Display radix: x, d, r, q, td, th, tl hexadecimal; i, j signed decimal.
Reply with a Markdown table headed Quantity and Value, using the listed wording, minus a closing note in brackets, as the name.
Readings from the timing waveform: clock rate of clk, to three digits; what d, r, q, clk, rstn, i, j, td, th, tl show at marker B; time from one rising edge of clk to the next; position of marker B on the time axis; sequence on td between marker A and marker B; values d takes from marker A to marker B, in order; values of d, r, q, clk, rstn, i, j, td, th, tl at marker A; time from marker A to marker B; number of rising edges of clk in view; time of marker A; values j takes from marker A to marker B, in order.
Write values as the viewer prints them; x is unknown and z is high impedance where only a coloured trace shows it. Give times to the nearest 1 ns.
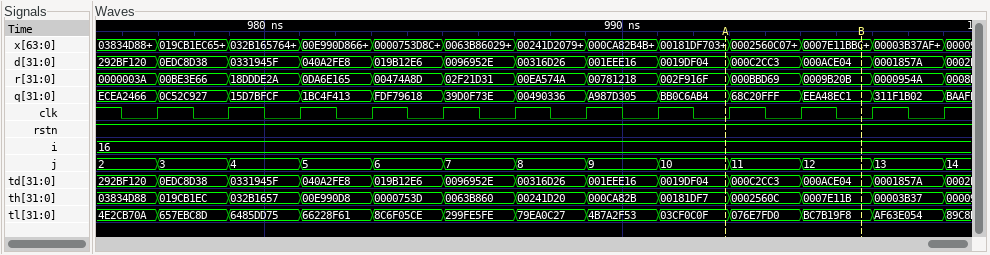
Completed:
| Quantity | Value |
|---|---|
| clock rate of clk, to three digits | 500 MHz |
| what d, r, q, clk, rstn, i, j, td, th, tl show at marker B | d=000ACE04, r=0009B20B, q=EEA48EC1, clk=0, rstn=1, i=16, j=12, td=000ACE04, th=0007E11B, tl=BC7B19F8 |
| time from one rising edge of clk to the next | 2 ns |
| position of marker B on the time axis | 997 ns |
| sequence on td between marker A and marker B | 0019DF04, 000C2CC3, 000ACE04 |
| values d takes from marker A to marker B, in order | 0019DF04, 000C2CC3, 000ACE04 |
| values of d, r, q, clk, rstn, i, j, td, th, tl at marker A | d=0019DF04, r=002F916F, q=BB0C6AB4, clk=0, rstn=1, i=16, j=10, td=0019DF04, th=00181DF7, tl=03CF0C0F |
| time from marker A to marker B | 4 ns |
| number of rising edges of clk in view | 12 |
| time of marker A | 993 ns |
| values j takes from marker A to marker B, in order | 10, 11, 12 |
